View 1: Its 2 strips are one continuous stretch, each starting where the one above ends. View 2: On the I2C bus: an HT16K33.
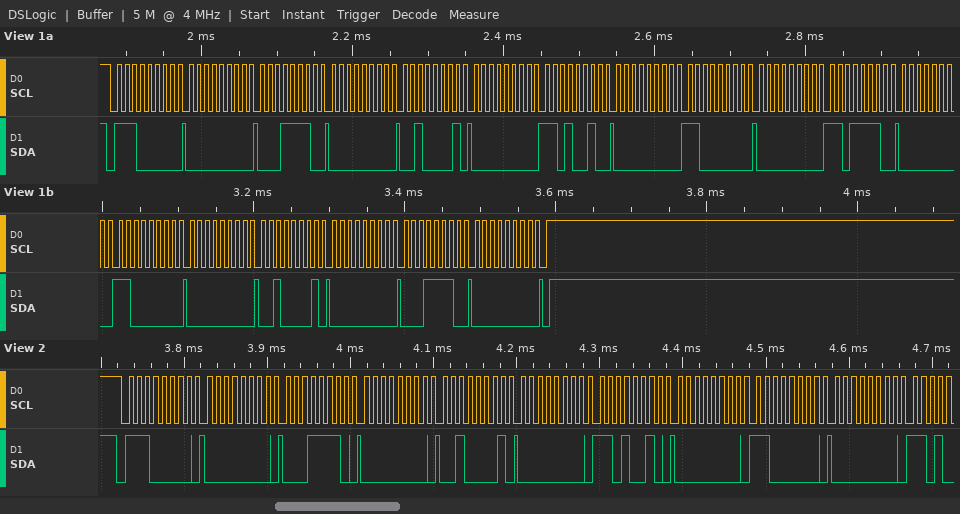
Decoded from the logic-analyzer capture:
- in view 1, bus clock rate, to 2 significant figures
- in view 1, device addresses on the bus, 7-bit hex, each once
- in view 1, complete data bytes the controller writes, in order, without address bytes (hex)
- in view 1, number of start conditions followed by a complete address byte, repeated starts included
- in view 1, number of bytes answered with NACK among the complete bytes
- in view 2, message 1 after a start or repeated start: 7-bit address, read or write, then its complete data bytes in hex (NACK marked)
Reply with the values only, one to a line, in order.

100 kHz
0x70
00 1E 00 21 00 D2 00 C0 00 DE 00 C0 00 21 00 1E 00
1
0
0x70 write: 00 1E 00 21 00 D2 00 C0 00
